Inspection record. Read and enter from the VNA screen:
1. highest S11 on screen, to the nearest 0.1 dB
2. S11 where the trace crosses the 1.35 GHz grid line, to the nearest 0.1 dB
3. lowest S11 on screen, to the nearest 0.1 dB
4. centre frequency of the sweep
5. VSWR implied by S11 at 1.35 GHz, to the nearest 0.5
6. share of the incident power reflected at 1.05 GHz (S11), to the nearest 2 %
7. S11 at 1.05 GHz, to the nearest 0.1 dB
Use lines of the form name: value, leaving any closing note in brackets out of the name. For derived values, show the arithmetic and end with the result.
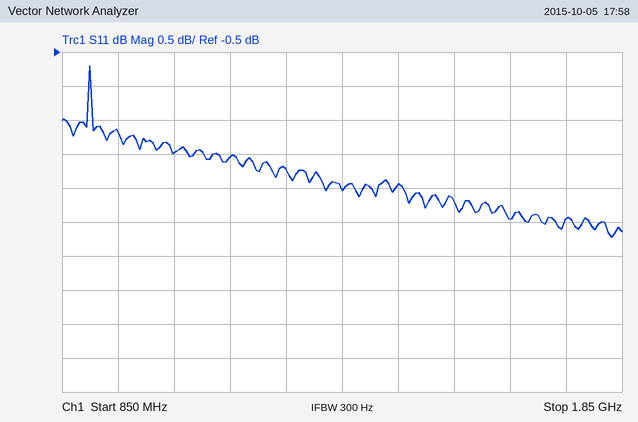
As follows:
highest S11 on screen, to the nearest 0.1 dB: -0.7 dB
S11 where the trace crosses the 1.35 GHz grid line, to the nearest 0.1 dB: -2.5 dB
lowest S11 on screen, to the nearest 0.1 dB: -3.2 dB
centre frequency of the sweep: 1.35 GHz
VSWR implied by S11 at 1.35 GHz, to the nearest 0.5: |Γ| = 10^(-2.5/20) = 0.7499; VSWR = (1 + 0.7499)/(1 − 0.7499) ≈ 7.0
share of the incident power reflected at 1.05 GHz (S11), to the nearest 2 %: 10^(-2/10) ≈ 63.1 %, so 64 % to the nearest 2 %
S11 at 1.05 GHz, to the nearest 0.1 dB: -2.0 dB
